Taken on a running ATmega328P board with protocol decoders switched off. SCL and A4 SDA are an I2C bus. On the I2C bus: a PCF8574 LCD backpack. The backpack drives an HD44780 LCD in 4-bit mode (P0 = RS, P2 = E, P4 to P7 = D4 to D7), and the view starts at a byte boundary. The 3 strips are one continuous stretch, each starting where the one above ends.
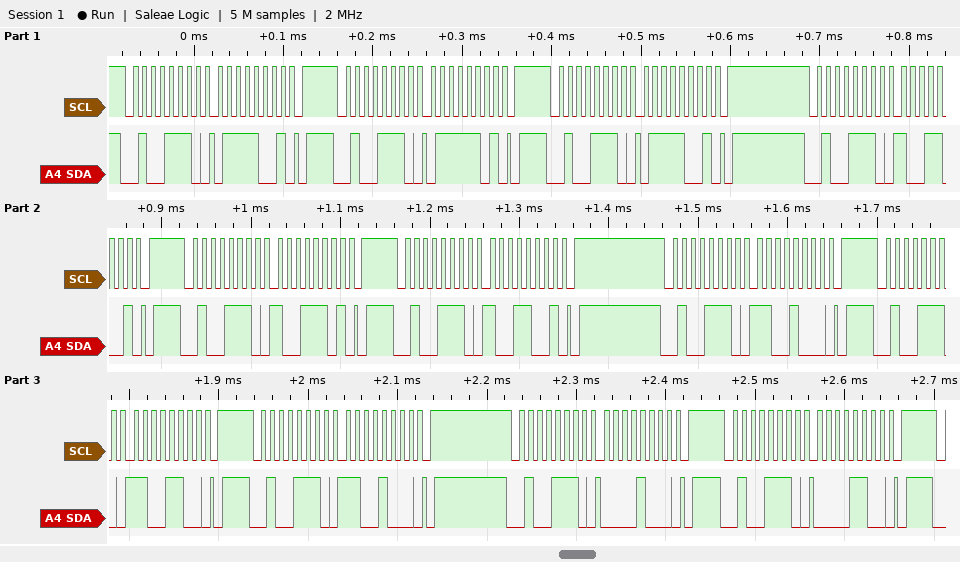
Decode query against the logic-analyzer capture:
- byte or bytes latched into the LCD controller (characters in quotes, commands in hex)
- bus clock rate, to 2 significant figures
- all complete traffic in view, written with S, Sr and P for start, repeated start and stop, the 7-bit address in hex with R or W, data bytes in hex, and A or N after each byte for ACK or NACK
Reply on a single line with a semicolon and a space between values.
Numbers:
'y'; 100 kHz; S 27W A 79 A P S 27W A 7D A P S 27W A 79 A P S 27W A 99 A P S 27W A 9D A P S 27W A 99 A P S 27W A C8 A P S 27W A CC A P S 27W A C8 A P S 27W A 08 A P S 27W A 0C A P
